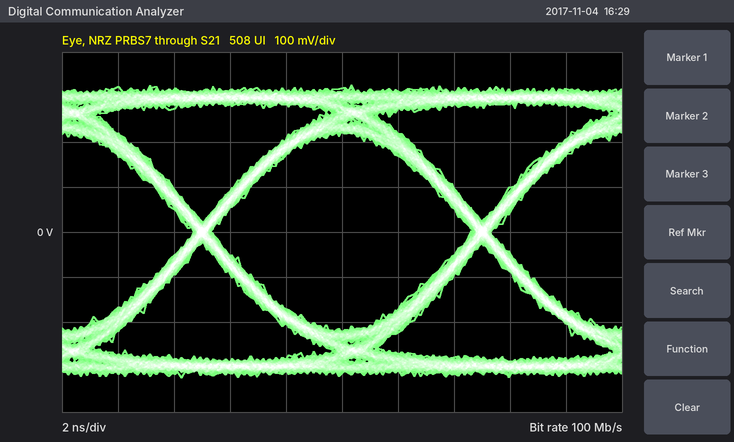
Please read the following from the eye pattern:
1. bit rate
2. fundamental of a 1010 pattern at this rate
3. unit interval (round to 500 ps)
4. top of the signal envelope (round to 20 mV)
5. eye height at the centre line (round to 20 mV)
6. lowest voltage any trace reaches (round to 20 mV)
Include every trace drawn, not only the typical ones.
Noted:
100 Mb/s
50 MHz
10.0 ns
320 mV
440 mV
-320 mV
